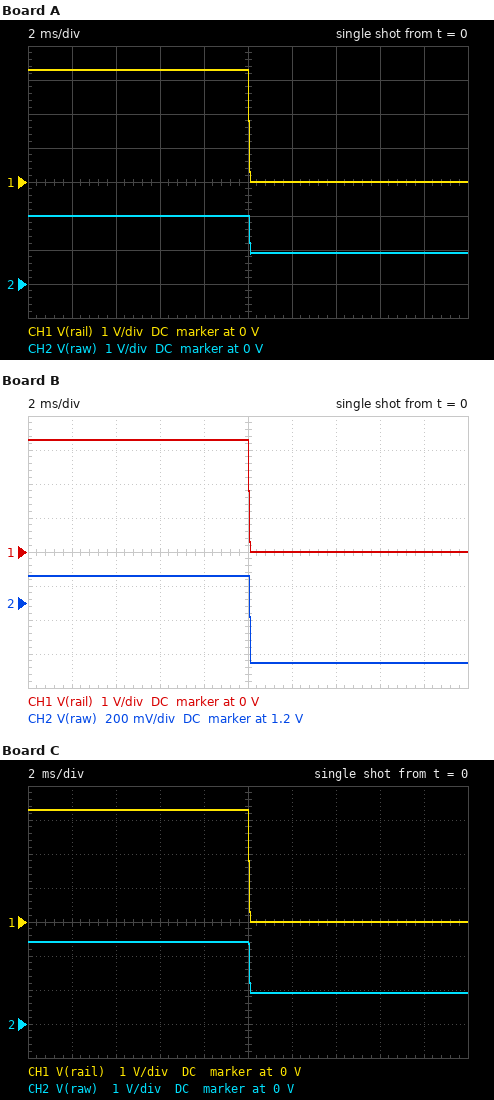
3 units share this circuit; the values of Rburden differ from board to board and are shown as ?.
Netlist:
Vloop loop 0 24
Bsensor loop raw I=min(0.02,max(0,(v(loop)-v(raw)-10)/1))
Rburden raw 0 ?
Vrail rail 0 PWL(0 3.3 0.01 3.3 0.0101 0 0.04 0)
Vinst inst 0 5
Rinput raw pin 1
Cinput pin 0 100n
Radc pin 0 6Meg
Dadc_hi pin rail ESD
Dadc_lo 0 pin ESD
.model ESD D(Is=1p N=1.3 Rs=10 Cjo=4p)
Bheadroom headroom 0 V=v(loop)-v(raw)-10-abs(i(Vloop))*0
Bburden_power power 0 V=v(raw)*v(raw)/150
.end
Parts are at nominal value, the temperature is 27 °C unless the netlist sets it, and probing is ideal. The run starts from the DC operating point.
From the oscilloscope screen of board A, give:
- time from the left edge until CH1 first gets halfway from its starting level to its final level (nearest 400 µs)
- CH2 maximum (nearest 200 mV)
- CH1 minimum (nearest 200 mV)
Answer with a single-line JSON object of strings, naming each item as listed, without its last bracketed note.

{"time from the left edge until CH1 first gets halfway from its starting level to its final level": "10.0 ms", "CH2 maximum": "2.0 V", "CH1 minimum": "0 V"}
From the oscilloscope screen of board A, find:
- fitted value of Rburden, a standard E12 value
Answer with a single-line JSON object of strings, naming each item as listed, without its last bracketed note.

{"fitted value of Rburden, a standard E12 value": "100 Ω"}
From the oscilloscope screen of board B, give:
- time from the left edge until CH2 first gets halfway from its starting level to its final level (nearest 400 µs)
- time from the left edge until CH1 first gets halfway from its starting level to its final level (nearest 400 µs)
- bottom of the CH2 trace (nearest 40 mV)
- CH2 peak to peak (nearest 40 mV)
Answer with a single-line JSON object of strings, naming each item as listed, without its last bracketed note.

{"time from the left edge until CH2 first gets halfway from its starting level to its final level": "10.0 ms", "time from the left edge until CH1 first gets halfway from its starting level to its final level": "10.0 ms", "bottom of the CH2 trace": "840 mV", "CH2 peak to peak": "520 mV"}
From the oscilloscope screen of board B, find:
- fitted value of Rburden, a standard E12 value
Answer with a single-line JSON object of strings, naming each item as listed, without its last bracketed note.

{"fitted value of Rburden, a standard E12 value": "68 Ω"}
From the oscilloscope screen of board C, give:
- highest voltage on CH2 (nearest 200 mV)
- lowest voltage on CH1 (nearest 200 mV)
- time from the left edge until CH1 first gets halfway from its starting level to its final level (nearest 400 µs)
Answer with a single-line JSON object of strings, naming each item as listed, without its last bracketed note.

{"highest voltage on CH2": "2.4 V", "lowest voltage on CH1": "0 V", "time from the left edge until CH1 first gets halfway from its starting level to its final level": "10.0 ms"}
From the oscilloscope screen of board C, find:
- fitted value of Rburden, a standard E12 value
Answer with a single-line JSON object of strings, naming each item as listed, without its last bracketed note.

{"fitted value of Rburden, a standard E12 value": "120 Ω"}
